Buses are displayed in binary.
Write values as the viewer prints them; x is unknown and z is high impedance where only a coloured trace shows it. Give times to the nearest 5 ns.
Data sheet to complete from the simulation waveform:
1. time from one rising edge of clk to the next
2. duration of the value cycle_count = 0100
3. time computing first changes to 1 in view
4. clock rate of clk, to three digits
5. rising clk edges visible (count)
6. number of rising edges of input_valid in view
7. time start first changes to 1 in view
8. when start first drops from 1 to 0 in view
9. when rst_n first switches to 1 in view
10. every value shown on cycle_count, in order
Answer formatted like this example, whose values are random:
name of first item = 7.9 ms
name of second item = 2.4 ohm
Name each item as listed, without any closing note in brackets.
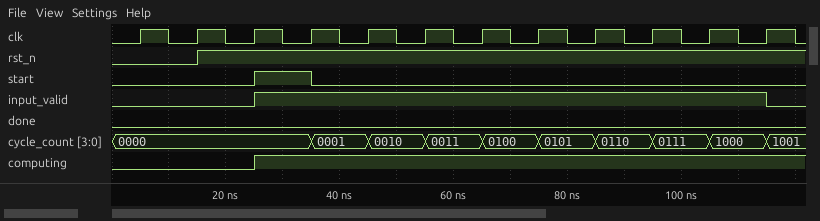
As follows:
time from one rising edge of clk to the next = 10 ns
duration of the value cycle_count = 0100 = 10 ns
time computing first changes to 1 in view = 25 ns
clock rate of clk, to three digits = 100 MHz
rising clk edges visible = 12
number of rising edges of input_valid in view = 1
time start first changes to 1 in view = 25 ns
when start first drops from 1 to 0 in view = 35 ns
when rst_n first switches to 1 in view = 15 ns
every value shown on cycle_count, in order = 0000, 0001, 0010, 0011, 0100, 0101, 0110, 0111, 1000, 1001
